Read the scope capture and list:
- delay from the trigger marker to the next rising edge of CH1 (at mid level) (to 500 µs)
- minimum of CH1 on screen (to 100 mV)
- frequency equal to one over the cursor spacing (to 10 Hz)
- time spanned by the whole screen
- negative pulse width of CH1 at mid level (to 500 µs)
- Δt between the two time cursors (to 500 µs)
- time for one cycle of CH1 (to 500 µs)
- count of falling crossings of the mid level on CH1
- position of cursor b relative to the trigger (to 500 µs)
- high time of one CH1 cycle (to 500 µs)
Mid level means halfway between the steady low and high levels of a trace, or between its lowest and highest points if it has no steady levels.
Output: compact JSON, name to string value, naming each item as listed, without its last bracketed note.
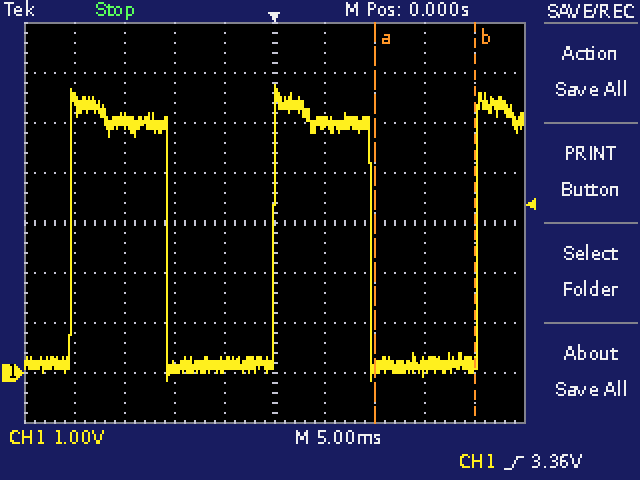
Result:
{"delay from the trigger marker to the next rising edge of CH1 (at mid level)": "20.5 ms", "minimum of CH1 on screen": "-200 mV", "frequency equal to one over the cursor spacing": "100 Hz", "time spanned by the whole screen": "50 ms", "negative pulse width of CH1 at mid level": "10.5 ms", "Δt between the two time cursors": "10.0 ms", "time for one cycle of CH1": "20.5 ms", "count of falling crossings of the mid level on CH1": "2", "position of cursor b relative to the trigger": "+20.0 ms", "high time of one CH1 cycle": "9.5 ms"}
